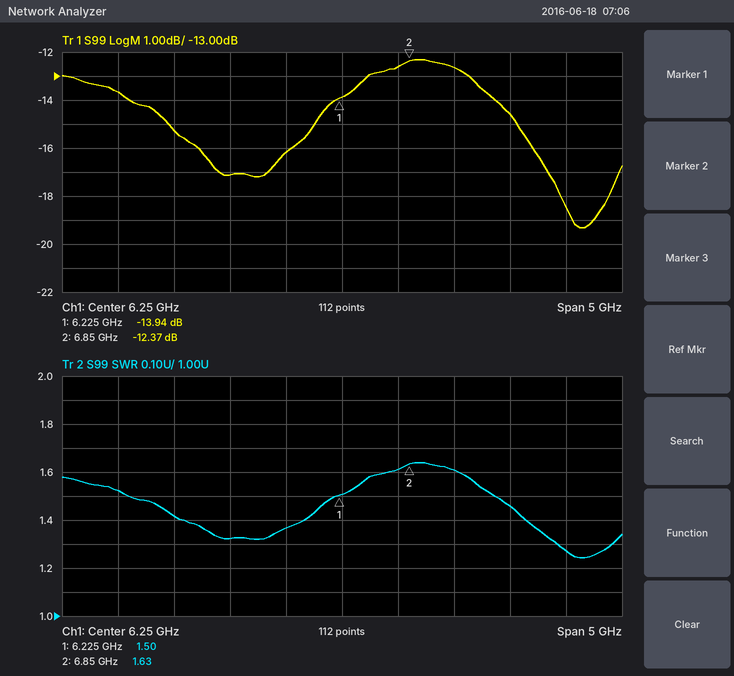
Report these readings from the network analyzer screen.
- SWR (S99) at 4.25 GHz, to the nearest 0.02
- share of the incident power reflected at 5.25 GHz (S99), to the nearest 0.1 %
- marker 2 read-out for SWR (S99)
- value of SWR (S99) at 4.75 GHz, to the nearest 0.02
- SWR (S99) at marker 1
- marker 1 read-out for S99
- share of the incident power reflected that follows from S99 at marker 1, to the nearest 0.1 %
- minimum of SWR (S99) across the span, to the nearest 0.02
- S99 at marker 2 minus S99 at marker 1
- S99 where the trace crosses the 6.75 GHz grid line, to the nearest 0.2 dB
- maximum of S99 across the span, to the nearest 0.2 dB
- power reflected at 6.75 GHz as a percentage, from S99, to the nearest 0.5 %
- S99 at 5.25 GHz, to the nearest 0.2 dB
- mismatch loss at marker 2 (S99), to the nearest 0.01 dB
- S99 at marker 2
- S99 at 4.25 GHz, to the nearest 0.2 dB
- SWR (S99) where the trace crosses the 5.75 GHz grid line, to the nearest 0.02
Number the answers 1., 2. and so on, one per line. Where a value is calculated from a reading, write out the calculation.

1. 1.52
2. 10^(-17.2/10) ≈ 1.9 %
3. 1.63
4. 1.42
5. 1.50
6. -13.94 dB
7. 10^(-13.94/10) ≈ 4.0 %
8. 1.24
9. -12.37 − (-13.94) = 1.57 dB
10. -12.6 dB
11. -12.4 dB
12. 10^(-12.6/10) ≈ 5.5 %
13. -17.2 dB
14. −10 log10(1 − 10^(-12.37/10)) ≈ 0.26 dB
15. -12.37 dB
16. -13.6 dB
17. 1.36
